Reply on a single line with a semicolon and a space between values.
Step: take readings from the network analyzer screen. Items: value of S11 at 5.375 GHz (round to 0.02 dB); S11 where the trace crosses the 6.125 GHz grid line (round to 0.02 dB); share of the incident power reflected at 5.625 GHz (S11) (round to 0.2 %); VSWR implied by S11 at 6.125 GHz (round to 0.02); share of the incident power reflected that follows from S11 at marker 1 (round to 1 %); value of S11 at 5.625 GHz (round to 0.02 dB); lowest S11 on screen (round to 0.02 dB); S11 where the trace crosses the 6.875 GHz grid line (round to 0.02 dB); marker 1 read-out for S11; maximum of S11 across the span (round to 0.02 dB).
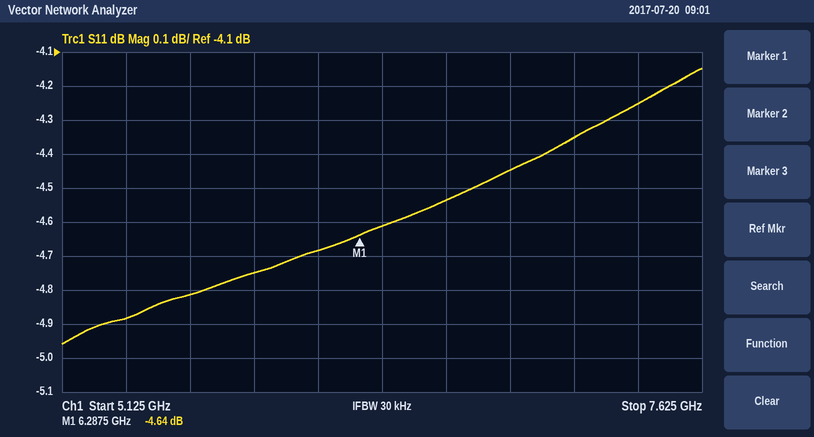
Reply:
-4.88 dB; -4.68 dB; 33.0 %; 3.80; 34 %; -4.82 dB; -4.96 dB; -4.44 dB; -4.64 dB; -4.14 dB
